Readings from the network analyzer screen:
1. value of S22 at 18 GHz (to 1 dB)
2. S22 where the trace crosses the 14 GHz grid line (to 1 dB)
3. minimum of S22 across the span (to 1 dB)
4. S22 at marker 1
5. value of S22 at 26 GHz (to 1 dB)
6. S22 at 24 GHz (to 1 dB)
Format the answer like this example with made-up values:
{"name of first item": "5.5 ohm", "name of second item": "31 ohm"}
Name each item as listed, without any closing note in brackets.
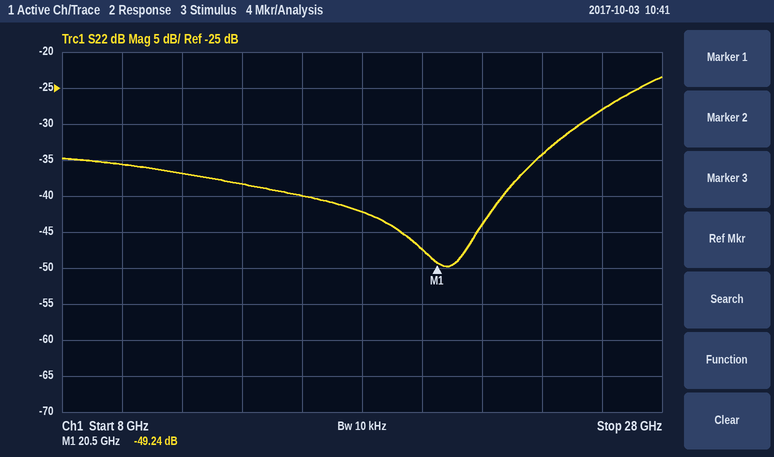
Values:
{"value of S22 at 18 GHz": "-42 dB", "S22 where the trace crosses the 14 GHz grid line": "-38 dB", "minimum of S22 across the span": "-50 dB", "S22 at marker 1": "-49.24 dB", "value of S22 at 26 GHz": "-28 dB", "S22 at 24 GHz": "-34 dB"}
